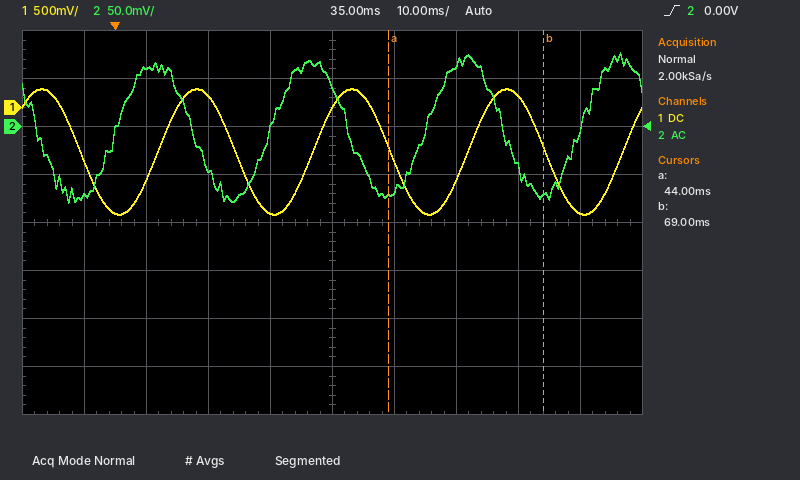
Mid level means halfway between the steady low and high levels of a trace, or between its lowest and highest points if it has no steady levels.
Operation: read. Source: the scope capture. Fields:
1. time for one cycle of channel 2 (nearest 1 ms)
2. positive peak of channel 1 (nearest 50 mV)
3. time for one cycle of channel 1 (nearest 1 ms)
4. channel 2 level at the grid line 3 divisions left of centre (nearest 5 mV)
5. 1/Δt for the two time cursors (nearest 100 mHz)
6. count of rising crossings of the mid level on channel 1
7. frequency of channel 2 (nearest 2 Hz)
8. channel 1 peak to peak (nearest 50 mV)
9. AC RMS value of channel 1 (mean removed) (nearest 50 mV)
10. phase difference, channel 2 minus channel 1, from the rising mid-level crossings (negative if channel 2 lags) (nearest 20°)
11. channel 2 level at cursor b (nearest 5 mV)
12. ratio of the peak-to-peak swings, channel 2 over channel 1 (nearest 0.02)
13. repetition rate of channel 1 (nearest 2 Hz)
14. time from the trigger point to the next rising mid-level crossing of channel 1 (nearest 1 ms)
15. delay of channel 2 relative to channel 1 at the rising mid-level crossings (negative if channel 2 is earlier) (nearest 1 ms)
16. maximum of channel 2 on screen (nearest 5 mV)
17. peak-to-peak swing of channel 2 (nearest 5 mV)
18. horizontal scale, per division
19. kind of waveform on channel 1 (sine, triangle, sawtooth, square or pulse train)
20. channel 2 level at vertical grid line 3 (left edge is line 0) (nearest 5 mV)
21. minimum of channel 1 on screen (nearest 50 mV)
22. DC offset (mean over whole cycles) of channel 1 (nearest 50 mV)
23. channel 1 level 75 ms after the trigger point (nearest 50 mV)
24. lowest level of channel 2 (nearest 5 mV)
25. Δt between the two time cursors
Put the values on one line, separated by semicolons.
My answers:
25 ms; 200 mV; 25 ms; 60 mV; 40.0 Hz; 4; 40 Hz; 1.30 V; 450 mV; +100°; -70 mV; 0.12; 40 Hz; 7 ms; -7 ms; 75 mV; 155 mV; 10 ms; sine; -45 mV; -1.10 V; -450 mV; -1.10 V; -80 mV; 25 ms
